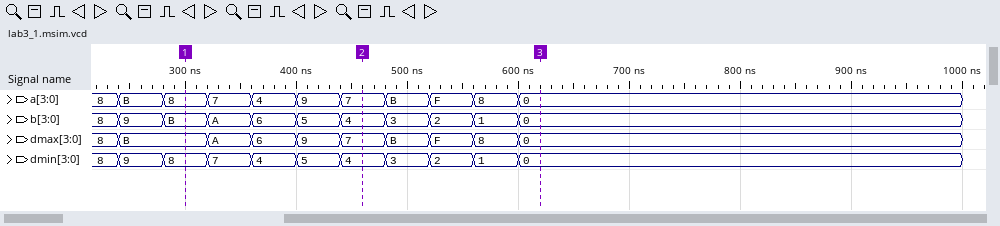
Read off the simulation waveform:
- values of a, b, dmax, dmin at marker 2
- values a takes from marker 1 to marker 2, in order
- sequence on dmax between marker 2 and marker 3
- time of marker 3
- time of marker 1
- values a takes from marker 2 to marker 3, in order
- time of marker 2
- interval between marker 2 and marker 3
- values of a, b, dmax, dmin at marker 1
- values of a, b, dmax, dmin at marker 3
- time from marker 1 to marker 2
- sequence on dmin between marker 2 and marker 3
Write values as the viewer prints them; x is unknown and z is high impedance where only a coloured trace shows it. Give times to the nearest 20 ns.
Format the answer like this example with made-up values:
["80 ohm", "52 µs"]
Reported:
["a=7, b=4, dmax=7, dmin=4", "8, 7, 4, 9, 7", "7, B, F, 8, 0", "620 ns", "300 ns", "7, B, F, 8, 0", "460 ns", "160 ns", "a=8, b=B, dmax=B, dmin=8", "a=0, b=0, dmax=0, dmin=0", "160 ns", "4, 3, 2, 1, 0"]
